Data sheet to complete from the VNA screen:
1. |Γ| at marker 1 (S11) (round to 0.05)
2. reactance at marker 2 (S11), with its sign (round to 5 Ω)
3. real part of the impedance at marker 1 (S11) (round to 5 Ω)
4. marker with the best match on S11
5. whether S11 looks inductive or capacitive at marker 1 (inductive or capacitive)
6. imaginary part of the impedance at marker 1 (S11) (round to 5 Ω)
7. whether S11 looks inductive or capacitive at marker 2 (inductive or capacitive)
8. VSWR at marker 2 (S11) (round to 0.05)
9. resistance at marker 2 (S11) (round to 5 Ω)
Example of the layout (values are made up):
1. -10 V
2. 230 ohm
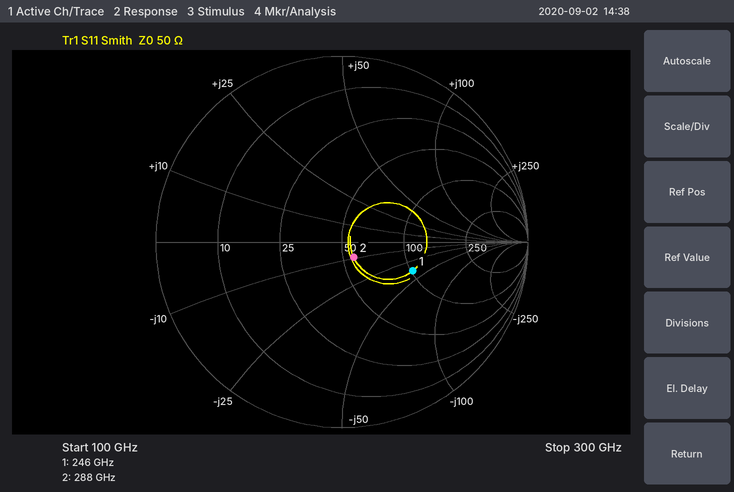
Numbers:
1. 0.40
2. -10 Ω
3. 100 Ω
4. marker 2
5. capacitive
6. -40 Ω
7. capacitive
8. 1.25
9. 55 Ω
